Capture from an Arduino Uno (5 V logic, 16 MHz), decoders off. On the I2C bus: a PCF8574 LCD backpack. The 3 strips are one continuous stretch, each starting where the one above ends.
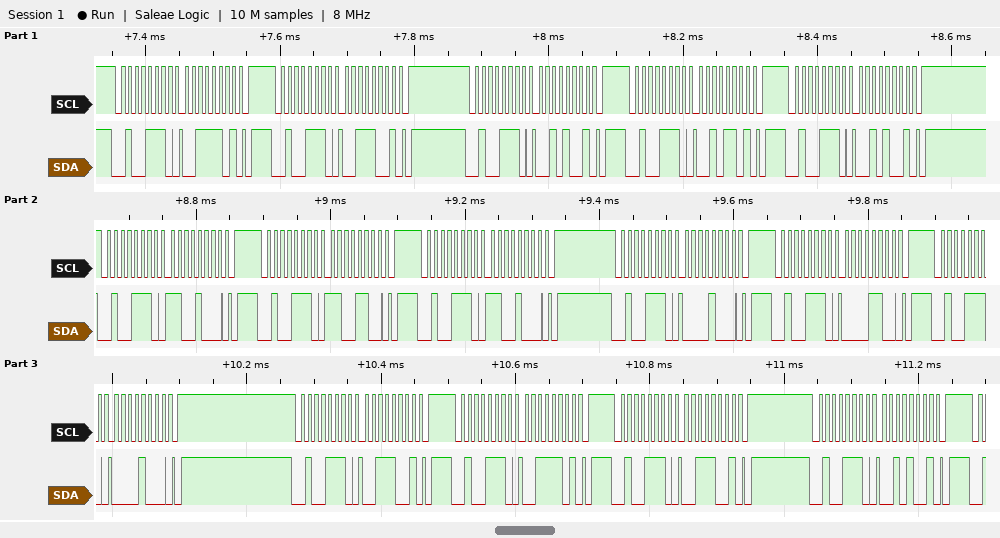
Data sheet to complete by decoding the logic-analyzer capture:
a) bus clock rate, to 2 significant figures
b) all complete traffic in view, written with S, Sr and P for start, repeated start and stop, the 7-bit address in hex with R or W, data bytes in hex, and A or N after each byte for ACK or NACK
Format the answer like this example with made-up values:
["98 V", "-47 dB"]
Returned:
["100 kHz", "S 27W A 3D A P S 27W A 39 A P S 27W A 29 A P S 27W A 2D A P S 27W A 29 A P S 27W A C8 A P S 27W A CC A P S 27W A C8 A P S 27W A 08 A P S 27W A 0C A P S 27W A 08 A P S 27W A 39 A P S 27W A 3D A P S 27W A 39 A P S 27W A 29 A P"]
